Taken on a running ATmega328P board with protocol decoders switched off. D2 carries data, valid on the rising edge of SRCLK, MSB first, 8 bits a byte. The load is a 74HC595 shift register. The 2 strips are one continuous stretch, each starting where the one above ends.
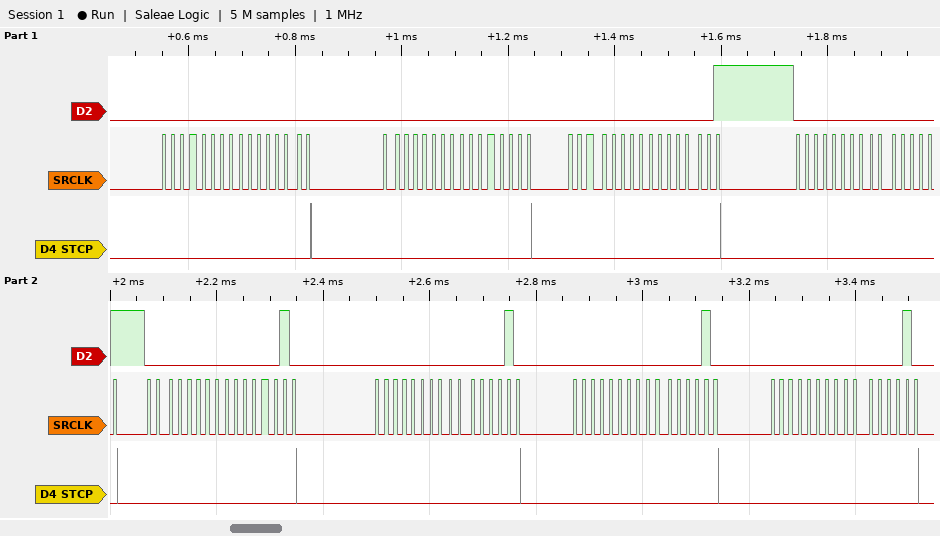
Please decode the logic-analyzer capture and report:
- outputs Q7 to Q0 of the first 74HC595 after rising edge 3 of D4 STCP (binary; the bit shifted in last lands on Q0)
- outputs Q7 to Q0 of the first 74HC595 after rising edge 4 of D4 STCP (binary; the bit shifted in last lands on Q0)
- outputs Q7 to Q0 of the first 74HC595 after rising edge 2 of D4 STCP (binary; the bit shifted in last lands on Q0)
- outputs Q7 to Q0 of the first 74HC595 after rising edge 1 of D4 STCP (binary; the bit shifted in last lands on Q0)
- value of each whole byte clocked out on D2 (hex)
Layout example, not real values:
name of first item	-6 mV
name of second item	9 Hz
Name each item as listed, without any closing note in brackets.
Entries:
outputs Q7 to Q0 of the first 74HC595 after rising edge 3 of D4 STCP	00000001
outputs Q7 to Q0 of the first 74HC595 after rising edge 4 of D4 STCP	00000001
outputs Q7 to Q0 of the first 74HC595 after rising edge 2 of D4 STCP	00000000
outputs Q7 to Q0 of the first 74HC595 after rising edge 1 of D4 STCP	00000000
value of each whole byte clocked out on D2	00 00 00 00 00 01 00 01 00 02 00 02 00 02 00 02
